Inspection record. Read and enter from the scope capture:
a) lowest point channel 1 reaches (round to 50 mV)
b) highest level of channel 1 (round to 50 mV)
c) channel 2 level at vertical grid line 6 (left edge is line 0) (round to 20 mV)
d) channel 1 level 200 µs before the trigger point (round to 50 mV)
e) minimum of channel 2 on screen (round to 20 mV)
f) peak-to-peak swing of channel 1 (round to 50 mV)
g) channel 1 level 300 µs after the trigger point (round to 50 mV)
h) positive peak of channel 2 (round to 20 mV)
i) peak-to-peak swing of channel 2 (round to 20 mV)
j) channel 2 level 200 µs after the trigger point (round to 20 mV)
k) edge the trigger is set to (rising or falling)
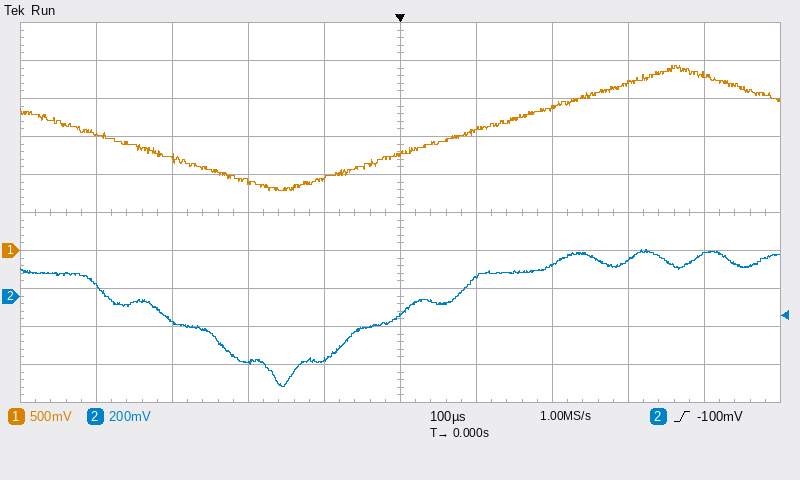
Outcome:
800 mV
2.45 V
100 mV
900 mV
-480 mV
1.65 V
2.20 V
240 mV
720 mV
160 mV
rising
